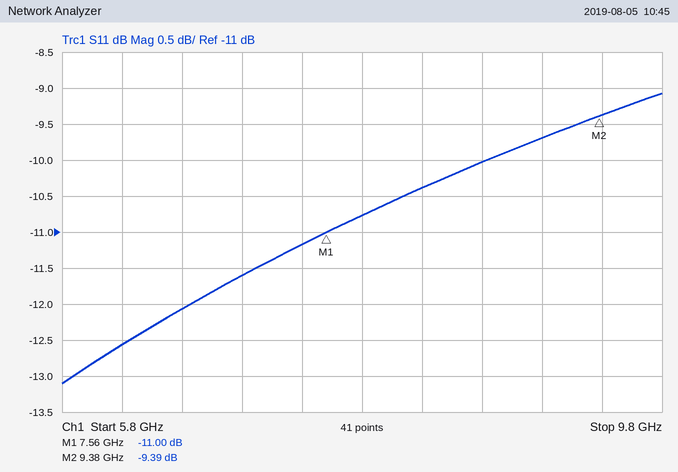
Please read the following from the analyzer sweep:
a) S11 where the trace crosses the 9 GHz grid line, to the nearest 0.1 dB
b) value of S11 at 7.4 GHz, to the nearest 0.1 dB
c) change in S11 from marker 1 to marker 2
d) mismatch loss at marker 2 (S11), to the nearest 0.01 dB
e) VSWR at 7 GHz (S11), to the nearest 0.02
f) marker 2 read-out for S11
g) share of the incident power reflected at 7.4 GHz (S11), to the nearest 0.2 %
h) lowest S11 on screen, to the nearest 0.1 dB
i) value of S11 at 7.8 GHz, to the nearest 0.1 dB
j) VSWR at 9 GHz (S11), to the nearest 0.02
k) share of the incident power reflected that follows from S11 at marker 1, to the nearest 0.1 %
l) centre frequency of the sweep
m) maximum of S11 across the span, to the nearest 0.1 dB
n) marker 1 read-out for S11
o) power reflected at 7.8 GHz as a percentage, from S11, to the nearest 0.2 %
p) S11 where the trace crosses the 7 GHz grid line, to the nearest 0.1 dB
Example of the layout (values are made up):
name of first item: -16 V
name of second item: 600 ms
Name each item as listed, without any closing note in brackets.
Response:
S11 where the trace crosses the 9 GHz grid line, to the nearest 0.1 dB: -9.7 dB
value of S11 at 7.4 GHz, to the nearest 0.1 dB: -11.2 dB
change in S11 from marker 1 to marker 2: 1.61 dB
mismatch loss at marker 2 (S11), to the nearest 0.01 dB: 0.53 dB
VSWR at 7 GHz (S11), to the nearest 0.02: 1.72
marker 2 read-out for S11: -9.39 dB
share of the incident power reflected at 7.4 GHz (S11), to the nearest 0.2 %: 7.6 %
lowest S11 on screen, to the nearest 0.1 dB: -13.1 dB
value of S11 at 7.8 GHz, to the nearest 0.1 dB: -10.8 dB
VSWR at 9 GHz (S11), to the nearest 0.02: 1.98
share of the incident power reflected that follows from S11 at marker 1, to the nearest 0.1 %: 7.9 %
centre frequency of the sweep: 7.8 GHz
maximum of S11 across the span, to the nearest 0.1 dB: -9.1 dB
marker 1 read-out for S11: -11.00 dB
power reflected at 7.8 GHz as a percentage, from S11, to the nearest 0.2 %: 8.4 %
S11 where the trace crosses the 7 GHz grid line, to the nearest 0.1 dB: -11.6 dB
